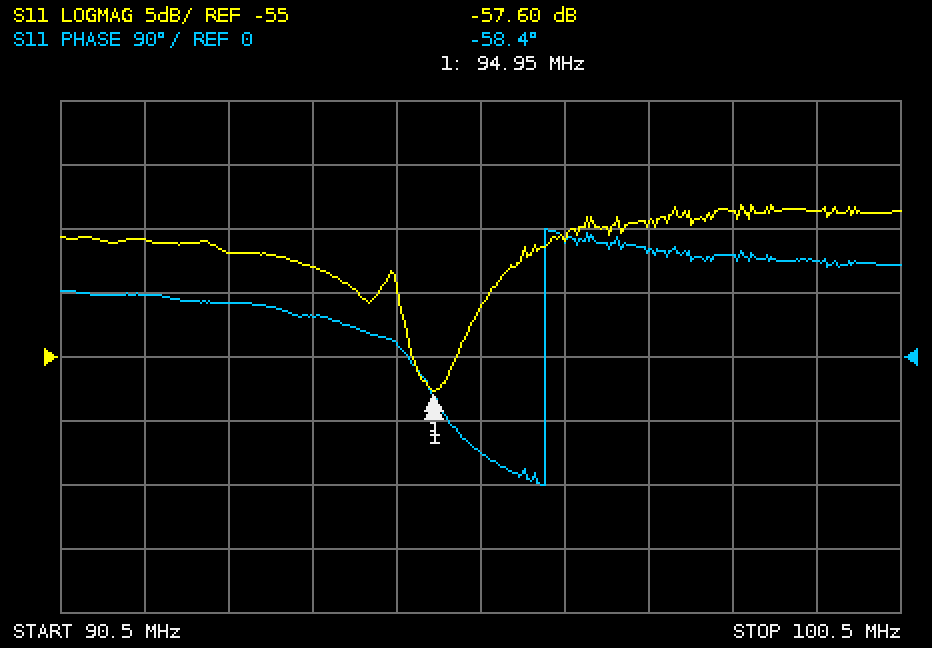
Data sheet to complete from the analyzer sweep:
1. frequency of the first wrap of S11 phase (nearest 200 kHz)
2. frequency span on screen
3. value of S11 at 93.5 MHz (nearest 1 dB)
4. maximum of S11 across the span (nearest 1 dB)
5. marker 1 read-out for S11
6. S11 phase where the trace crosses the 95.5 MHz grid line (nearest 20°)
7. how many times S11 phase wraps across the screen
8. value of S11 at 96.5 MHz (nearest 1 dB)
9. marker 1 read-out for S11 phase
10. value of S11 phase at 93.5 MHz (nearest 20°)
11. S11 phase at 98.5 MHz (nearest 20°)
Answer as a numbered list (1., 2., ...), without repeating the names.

1. 96.2 MHz
2. 10 MHz
3. -48 dB
4. -43 dB
5. -57.60 dB
6. -140°
7. 1
8. -46 dB
9. -58.4°
10. 60°
11. 140°
